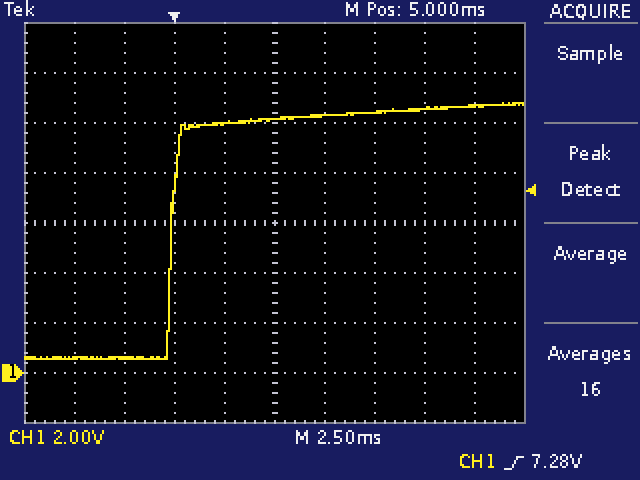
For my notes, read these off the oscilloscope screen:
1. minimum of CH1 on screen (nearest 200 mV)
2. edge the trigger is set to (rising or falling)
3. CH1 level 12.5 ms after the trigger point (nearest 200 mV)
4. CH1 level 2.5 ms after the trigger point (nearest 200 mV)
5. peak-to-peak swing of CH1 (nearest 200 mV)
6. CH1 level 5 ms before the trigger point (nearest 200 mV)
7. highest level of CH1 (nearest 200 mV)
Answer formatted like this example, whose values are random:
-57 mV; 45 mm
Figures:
600 mV; rising; 10.6 V; 10.0 V; 10.2 V; 600 mV; 10.8 V
